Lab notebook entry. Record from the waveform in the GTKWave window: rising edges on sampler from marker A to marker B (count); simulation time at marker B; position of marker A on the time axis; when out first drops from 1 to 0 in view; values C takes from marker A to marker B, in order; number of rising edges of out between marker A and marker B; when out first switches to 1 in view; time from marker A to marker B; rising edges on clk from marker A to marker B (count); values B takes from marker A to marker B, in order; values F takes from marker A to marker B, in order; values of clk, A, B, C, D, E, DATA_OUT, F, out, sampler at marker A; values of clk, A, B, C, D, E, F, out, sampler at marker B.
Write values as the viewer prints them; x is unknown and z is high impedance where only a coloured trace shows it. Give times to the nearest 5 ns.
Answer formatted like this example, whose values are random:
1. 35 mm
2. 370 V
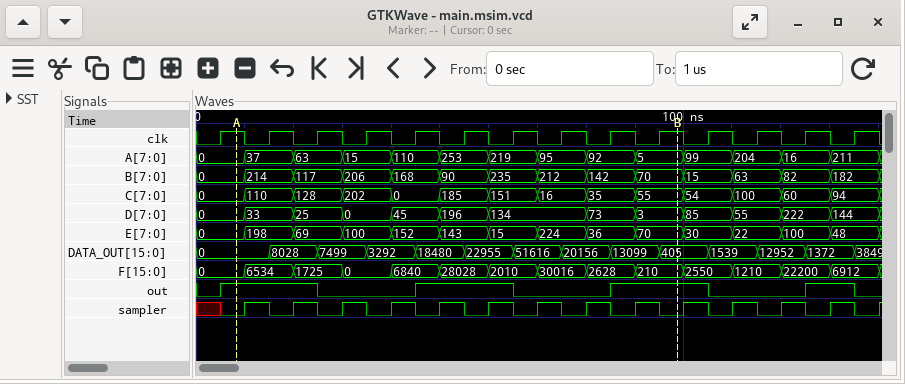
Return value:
1. 9
2. 100 ns
3. 10 ns
4. 25 ns
5. 0, 110, 128, 202, 0, 185, 151, 16, 35, 55
6. 2
7. 5 ns
8. 90 ns
9. 9
10. 0, 214, 117, 206, 168, 90, 235, 212, 142, 70
11. 0, 6534, 1725, 0, 6840, 28028, 2010, 30016, 2628, 210
12. clk=1, A=0, B=0, C=0, D=0, E=0, DATA_OUT=0, F=0, out=1, sampler=0
13. clk=1, A=5, B=70, C=55, D=3, E=70, F=210, out=1, sampler=0
